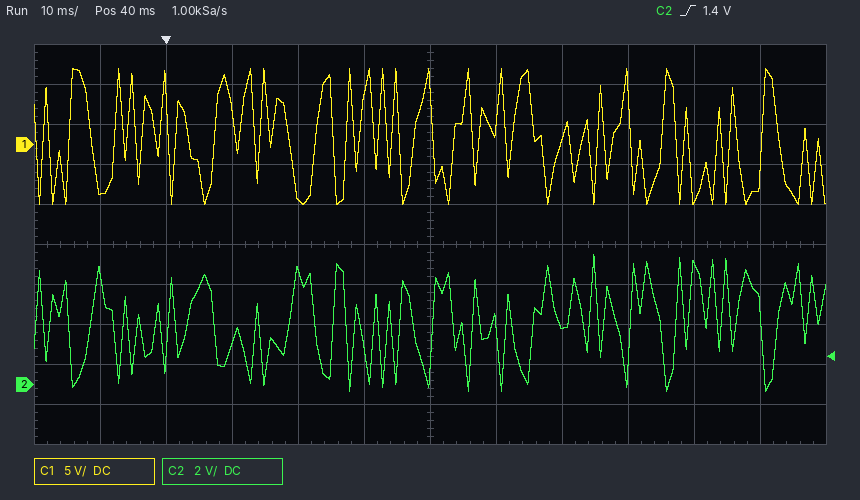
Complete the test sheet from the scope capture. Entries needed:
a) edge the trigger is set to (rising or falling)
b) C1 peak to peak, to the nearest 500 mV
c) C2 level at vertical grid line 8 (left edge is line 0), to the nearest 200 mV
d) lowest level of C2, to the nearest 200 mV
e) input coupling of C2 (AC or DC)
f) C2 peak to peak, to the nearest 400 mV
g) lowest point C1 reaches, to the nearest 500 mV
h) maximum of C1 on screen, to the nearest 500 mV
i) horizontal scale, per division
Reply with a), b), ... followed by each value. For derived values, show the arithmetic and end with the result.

a) rising
b) 9.5 V − (-7.5 V) = 17.0 V
c) 3.0 V
d) -400 mV
e) DC
f) 6.8 V
g) -7.5 V
h) 9.5 V
i) 10 ms
